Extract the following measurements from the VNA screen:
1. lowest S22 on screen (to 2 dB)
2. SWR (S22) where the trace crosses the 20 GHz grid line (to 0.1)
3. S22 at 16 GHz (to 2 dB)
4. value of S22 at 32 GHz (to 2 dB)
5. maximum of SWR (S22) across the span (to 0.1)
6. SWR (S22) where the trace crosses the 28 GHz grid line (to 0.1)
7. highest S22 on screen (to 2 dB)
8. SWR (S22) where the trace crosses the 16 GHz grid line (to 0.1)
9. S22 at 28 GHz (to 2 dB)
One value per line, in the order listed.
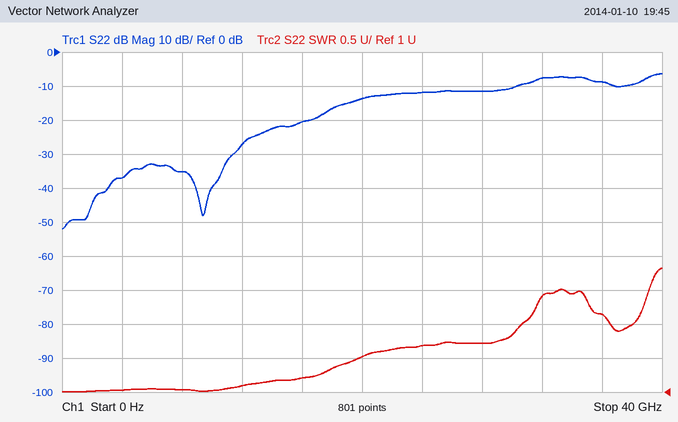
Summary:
-52 dB
1.5
-20 dB
-8 dB
2.8
1.7
-6 dB
1.2
-12 dB
